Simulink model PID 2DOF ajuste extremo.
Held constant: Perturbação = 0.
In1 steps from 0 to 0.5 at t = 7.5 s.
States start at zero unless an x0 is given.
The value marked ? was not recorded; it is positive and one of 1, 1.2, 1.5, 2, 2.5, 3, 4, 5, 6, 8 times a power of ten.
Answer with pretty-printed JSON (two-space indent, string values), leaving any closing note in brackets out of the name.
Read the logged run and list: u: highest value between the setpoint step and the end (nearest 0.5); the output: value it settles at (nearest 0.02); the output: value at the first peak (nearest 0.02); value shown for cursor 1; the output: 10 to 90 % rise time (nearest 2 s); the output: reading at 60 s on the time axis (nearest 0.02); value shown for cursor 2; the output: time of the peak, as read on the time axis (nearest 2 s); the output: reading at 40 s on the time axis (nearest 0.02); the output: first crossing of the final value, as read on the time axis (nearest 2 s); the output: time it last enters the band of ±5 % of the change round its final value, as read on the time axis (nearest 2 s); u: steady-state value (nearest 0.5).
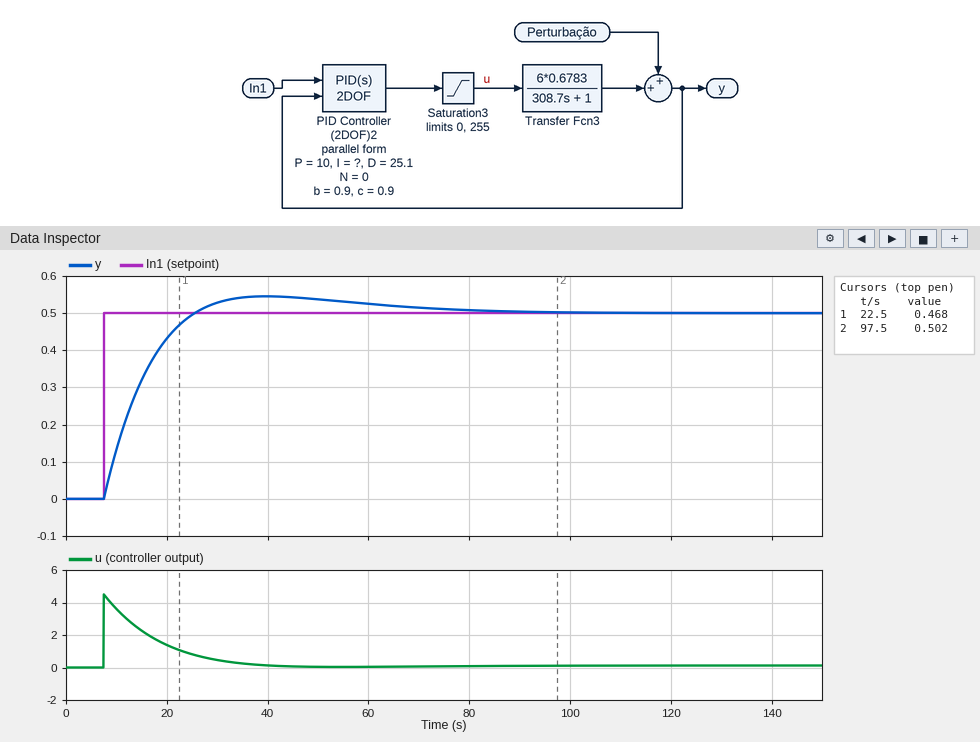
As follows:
{
  "u: highest value between the setpoint step and the end": "4.5",
  "the output: value it settles at": "0.50",
  "the output: value at the first peak": "0.54",
  "value shown for cursor 1": "0.468",
  "the output: 10 to 90 % rise time": "12 s",
  "the output: reading at 60 s on the time axis": "0.52",
  "value shown for cursor 2": "0.502",
  "the output: time of the peak, as read on the time axis": "40 s",
  "the output: reading at 40 s on the time axis": "0.54",
  "the output: first crossing of the final value, as read on the time axis": "26 s",
  "the output: time it last enters the band of ±5 % of the change round its final value, as read on the time axis": "60 s",
  "u: steady-state value": "0.0"
}
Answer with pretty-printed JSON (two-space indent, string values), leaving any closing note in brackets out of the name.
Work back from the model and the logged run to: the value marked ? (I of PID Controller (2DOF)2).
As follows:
{
  "the value marked ? (I of PID Controller (2DOF)2)": "0.4"
}
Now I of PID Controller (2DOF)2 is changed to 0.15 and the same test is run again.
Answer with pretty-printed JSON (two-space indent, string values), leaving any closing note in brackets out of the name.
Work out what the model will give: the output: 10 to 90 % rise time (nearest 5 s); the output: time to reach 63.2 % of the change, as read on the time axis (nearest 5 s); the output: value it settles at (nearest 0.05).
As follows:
{
  "the output: 10 to 90 % rise time": "20 s",
  "the output: time to reach 63.2 % of the change, as read on the time axis": "15 s",
  "the output: value it settles at": "0.50"
}
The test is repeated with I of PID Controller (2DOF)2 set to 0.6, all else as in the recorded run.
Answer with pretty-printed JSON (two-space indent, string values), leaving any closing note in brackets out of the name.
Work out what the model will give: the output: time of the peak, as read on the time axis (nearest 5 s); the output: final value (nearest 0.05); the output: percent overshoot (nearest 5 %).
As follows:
{
  "the output: time of the peak, as read on the time axis": "35 s",
  "the output: final value": "0.50",
  "the output: percent overshoot": "15 %"
}
